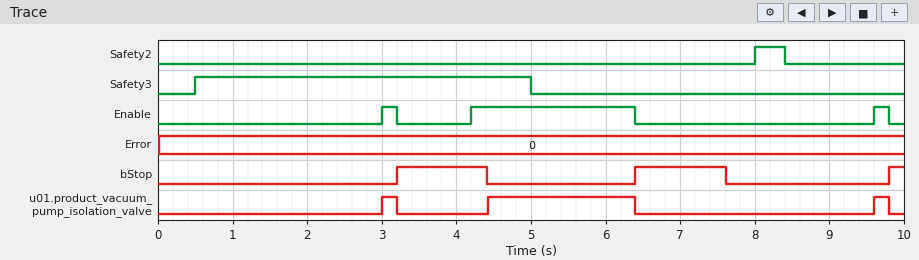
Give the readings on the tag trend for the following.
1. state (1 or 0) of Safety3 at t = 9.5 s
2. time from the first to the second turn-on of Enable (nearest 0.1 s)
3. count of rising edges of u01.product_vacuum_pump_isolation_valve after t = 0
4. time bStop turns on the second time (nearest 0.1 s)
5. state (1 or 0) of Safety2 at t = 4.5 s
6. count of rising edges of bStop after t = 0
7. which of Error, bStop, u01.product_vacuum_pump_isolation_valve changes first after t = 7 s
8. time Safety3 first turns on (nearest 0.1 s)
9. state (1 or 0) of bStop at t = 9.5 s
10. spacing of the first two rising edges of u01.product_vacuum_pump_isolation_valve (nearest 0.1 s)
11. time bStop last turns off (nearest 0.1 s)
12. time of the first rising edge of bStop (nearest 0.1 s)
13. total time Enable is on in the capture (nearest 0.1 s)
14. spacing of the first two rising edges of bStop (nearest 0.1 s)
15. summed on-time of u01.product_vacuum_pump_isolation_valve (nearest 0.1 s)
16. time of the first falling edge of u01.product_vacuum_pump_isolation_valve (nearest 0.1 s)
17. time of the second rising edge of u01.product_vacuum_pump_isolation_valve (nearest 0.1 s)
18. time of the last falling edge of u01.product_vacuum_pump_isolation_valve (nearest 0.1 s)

0
1.2 s
3
6.4 s
0
3
bStop
0.5 s
0
1.4 s
7.6 s
3.2 s
2.6 s
3.2 s
2.4 s
3.2 s
4.4 s
9.8 s
